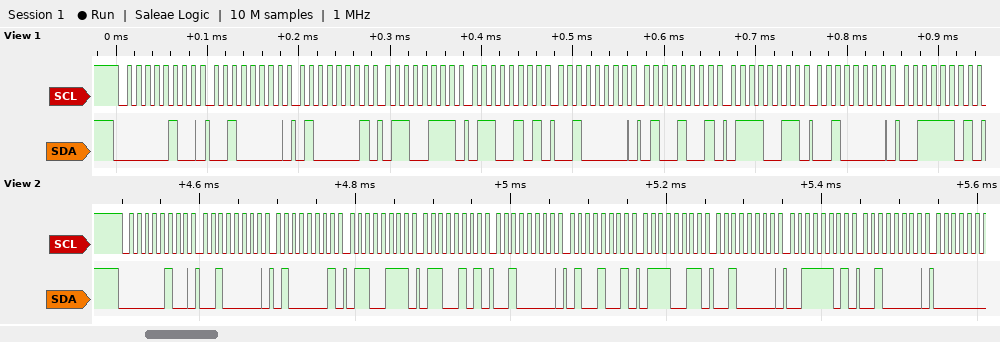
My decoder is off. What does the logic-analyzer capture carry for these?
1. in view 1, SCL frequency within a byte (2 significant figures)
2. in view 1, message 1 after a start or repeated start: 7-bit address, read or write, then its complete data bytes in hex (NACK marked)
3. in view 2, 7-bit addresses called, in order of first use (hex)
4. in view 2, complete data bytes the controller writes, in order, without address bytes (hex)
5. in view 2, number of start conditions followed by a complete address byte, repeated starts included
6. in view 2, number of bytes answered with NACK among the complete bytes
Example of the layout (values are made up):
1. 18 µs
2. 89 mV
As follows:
1. 100 kHz
2. 0x02 write: 20 41 67 65 20 49 73 20 3D
3. 0x02
4. 20 41 67 65 20 49 73 20 3D 20
5. 1
6. 0
